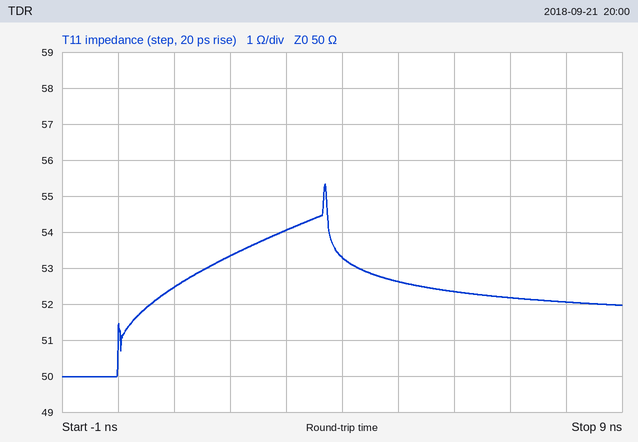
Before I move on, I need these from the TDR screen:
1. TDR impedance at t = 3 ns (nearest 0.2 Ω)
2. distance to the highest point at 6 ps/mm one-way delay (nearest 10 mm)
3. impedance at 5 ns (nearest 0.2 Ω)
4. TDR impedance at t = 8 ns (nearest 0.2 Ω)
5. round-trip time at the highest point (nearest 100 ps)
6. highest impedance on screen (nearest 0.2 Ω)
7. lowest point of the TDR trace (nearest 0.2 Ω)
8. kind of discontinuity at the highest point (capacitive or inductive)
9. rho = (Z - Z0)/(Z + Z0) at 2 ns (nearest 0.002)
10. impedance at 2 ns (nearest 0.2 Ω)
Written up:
54.0 Ω
310 mm
52.6 Ω
52.0 Ω
3.7 ns
55.4 Ω
50.0 Ω
inductive
+0.032
53.4 Ω
